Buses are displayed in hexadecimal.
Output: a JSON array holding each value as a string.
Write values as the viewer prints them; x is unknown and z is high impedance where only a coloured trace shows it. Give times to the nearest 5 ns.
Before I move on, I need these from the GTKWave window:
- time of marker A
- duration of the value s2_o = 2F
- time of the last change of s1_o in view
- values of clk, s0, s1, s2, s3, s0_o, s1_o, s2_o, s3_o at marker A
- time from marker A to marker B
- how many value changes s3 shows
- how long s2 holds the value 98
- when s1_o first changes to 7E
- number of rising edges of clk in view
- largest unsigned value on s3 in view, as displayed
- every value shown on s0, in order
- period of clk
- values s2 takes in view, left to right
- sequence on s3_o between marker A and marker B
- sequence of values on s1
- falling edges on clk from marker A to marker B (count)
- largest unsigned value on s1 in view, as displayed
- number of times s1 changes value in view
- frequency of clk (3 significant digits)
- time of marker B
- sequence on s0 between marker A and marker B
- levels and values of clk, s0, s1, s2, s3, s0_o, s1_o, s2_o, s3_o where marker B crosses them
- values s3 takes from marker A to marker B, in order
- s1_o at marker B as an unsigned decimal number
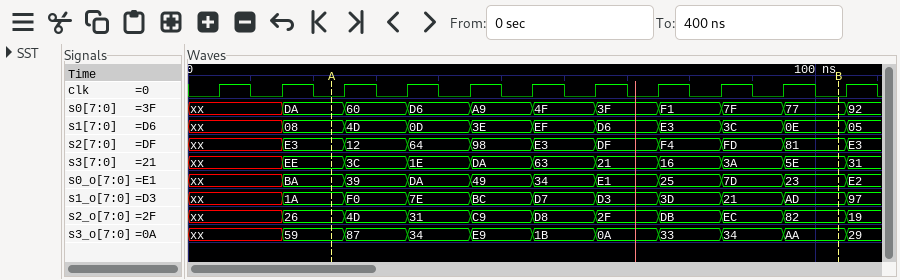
["25 ns", "10 ns", "105 ns", "clk=0, s0=DA, s1=08, s2=E3, s3=EE, s0_o=BA, s1_o=1A, s2_o=26, s3_o=59", "80 ns", "10", "10 ns", "35 ns", "11", "EE", "xx, DA, 60, D6, A9, 4F, 3F, F1, 7F, 77, 92", "10 ns", "xx, E3, 12, 64, 98, E3, DF, F4, FD, 81, E3", "59, 87, 34, E9, 1B, 0A, 33, 34, AA", "xx, 08, 4D, 0D, 3E, EF, D6, E3, 3C, 0E, 05", "8", "EF", "10", "100 MHz", "105 ns", "DA, 60, D6, A9, 4F, 3F, F1, 7F, 77", "clk=0, s0=77, s1=0E, s2=81, s3=5E, s0_o=23, s1_o=AD, s2_o=82, s3_o=AA", "EE, 3C, 1E, DA, 63, 21, 16, 3A, 5E", "173"]
